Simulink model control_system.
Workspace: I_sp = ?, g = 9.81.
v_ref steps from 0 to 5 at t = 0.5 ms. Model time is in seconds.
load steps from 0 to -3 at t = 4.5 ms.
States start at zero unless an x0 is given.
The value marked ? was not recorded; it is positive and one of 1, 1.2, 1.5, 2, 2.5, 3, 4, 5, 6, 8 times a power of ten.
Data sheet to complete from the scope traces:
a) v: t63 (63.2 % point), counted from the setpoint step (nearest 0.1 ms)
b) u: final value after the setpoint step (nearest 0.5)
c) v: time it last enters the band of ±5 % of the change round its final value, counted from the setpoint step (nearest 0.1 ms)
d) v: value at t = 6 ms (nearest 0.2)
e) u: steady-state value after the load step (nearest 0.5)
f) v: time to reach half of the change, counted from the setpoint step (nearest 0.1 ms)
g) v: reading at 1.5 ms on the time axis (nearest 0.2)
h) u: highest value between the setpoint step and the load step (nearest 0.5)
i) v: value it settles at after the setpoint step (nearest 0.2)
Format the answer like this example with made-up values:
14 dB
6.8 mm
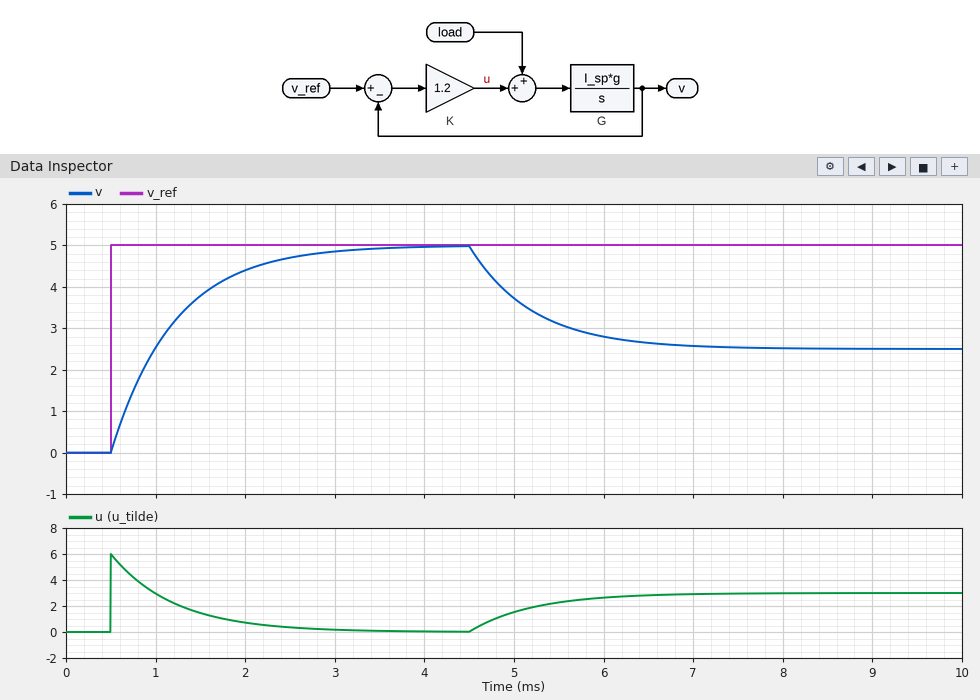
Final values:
0.7 ms
0.0
2.1 ms
2.8
3.0
0.5 ms
3.8
6.0
5.0
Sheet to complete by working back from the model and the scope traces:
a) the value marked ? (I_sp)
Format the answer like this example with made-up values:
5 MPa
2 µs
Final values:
120
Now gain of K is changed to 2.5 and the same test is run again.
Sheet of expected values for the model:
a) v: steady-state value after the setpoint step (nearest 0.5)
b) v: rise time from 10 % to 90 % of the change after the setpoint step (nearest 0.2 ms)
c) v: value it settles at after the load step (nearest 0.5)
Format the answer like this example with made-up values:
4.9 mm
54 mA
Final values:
5.0
0.8 ms
4.0
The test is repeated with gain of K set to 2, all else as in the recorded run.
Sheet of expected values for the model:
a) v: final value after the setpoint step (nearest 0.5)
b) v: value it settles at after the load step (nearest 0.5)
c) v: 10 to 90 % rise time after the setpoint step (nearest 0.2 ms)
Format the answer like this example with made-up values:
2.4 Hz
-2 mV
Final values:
5.0
3.5
1.0 ms
